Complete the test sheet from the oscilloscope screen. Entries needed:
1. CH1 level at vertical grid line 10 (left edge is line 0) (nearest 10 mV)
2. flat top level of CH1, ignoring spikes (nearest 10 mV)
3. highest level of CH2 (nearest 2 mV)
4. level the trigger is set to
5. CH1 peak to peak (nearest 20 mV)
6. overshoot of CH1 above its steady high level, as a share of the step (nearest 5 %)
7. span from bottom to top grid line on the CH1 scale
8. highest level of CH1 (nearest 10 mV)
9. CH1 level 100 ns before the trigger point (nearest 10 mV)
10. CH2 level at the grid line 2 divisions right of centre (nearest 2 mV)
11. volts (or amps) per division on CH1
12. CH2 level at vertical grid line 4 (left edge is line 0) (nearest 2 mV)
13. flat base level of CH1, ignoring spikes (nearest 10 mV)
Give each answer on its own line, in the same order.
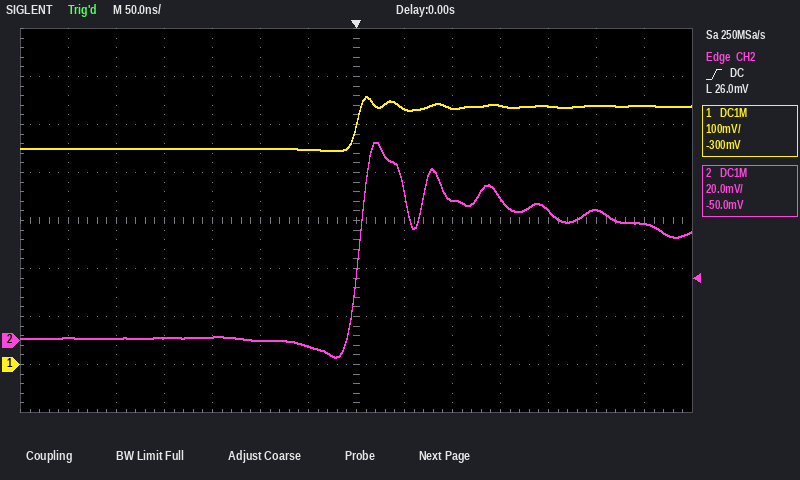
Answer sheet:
540 mV
540 mV
82 mV
26.0 mV
120 mV
25 %
800 mV
560 mV
450 mV
58 mV
100 mV
2 mV
450 mV
